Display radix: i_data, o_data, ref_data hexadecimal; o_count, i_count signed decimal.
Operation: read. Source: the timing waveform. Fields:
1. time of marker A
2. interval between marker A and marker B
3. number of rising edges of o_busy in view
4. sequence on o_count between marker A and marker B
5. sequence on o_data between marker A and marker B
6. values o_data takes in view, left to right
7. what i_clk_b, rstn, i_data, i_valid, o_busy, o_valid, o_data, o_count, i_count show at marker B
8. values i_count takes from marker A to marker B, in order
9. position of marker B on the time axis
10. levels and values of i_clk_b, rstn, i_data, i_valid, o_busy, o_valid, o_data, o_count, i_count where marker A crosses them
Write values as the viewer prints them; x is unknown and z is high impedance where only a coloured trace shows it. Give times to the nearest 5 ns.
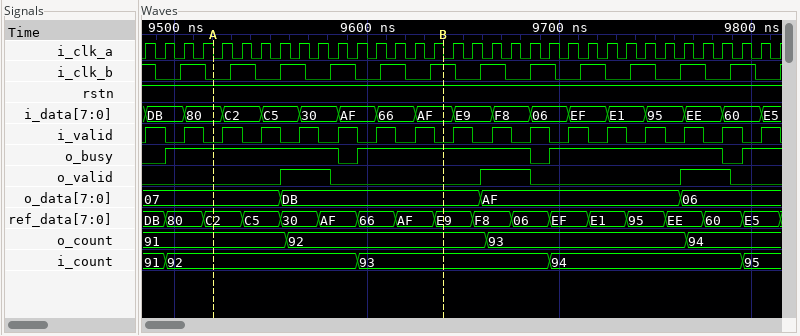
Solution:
9520 ns
120 ns
4
91, 92
07, DB
07, DB, AF, 06
i_clk_b=1, rstn=1, i_data=AF, i_valid=0, o_busy=1, o_valid=0, o_data=DB, o_count=92, i_count=93
92, 93
9640 ns
i_clk_b=0, rstn=1, i_data=80, i_valid=0, o_busy=1, o_valid=0, o_data=07, o_count=91, i_count=92
